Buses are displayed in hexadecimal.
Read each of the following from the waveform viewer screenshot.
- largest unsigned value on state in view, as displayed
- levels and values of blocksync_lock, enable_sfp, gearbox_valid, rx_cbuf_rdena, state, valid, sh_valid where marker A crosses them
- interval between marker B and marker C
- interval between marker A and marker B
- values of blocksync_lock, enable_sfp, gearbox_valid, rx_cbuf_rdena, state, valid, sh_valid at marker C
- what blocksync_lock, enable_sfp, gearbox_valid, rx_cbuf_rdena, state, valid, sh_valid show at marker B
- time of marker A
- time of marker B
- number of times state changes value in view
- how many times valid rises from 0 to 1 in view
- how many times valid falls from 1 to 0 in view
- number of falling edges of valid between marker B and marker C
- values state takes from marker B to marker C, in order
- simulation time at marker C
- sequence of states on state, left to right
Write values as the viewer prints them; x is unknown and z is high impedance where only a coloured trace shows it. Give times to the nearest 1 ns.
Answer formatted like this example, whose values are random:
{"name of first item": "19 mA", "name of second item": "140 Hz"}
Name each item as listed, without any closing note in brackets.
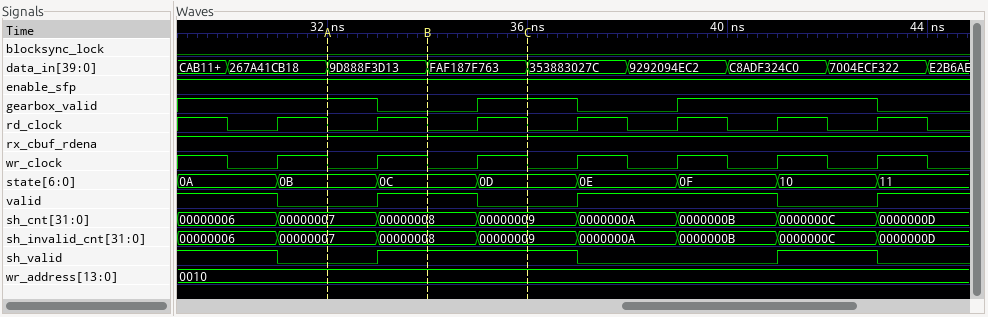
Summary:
{"largest unsigned value on state in view, as displayed": "11", "levels and values of blocksync_lock, enable_sfp, gearbox_valid, rx_cbuf_rdena, state, valid, sh_valid where marker A crosses them": "blocksync_lock=0, enable_sfp=1, gearbox_valid=1, rx_cbuf_rdena=1, state=0B, valid=0, sh_valid=0", "interval between marker B and marker C": "2 ns", "interval between marker A and marker B": "2 ns", "values of blocksync_lock, enable_sfp, gearbox_valid, rx_cbuf_rdena, state, valid, sh_valid at marker C": "blocksync_lock=0, enable_sfp=1, gearbox_valid=1, rx_cbuf_rdena=1, state=0D, valid=0, sh_valid=1", "what blocksync_lock, enable_sfp, gearbox_valid, rx_cbuf_rdena, state, valid, sh_valid show at marker B": "blocksync_lock=0, enable_sfp=1, gearbox_valid=0, rx_cbuf_rdena=1, state=0C, valid=1, sh_valid=1", "time of marker A": "32 ns", "time of marker B": "34 ns", "number of times state changes value in view": "7", "how many times valid rises from 0 to 1 in view": "3", "how many times valid falls from 1 to 0 in view": "3", "number of falling edges of valid between marker B and marker C": "1", "values state takes from marker B to marker C, in order": "0C, 0D", "simulation time at marker C": "36 ns", "sequence of states on state, left to right": "0A, 0B, 0C, 0D, 0E, 0F, 10, 11"}
